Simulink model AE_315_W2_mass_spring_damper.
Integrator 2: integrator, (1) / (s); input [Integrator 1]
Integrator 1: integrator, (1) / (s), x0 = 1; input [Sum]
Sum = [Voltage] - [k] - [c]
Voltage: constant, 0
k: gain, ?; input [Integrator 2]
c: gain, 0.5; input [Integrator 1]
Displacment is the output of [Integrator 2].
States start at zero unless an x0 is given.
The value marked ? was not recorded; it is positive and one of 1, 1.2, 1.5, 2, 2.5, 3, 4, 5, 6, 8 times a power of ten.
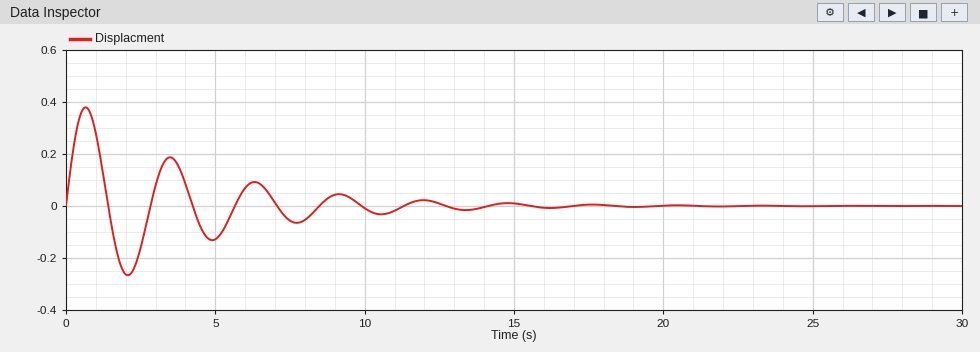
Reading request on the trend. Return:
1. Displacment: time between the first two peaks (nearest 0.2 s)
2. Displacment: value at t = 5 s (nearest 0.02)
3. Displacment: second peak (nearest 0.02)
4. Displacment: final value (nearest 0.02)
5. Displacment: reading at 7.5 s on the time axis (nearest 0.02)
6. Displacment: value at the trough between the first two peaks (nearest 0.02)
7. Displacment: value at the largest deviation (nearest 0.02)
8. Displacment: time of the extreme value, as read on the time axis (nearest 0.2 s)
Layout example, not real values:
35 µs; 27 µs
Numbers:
2.8 s; -0.12; 0.18; 0.00; -0.06; -0.26; 0.38; 0.6 s
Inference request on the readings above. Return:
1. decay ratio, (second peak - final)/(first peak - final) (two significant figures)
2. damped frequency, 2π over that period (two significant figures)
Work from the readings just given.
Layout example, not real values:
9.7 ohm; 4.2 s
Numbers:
0.47; 2.2 rad/s
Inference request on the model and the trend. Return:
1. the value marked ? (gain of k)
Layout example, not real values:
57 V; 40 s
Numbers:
5
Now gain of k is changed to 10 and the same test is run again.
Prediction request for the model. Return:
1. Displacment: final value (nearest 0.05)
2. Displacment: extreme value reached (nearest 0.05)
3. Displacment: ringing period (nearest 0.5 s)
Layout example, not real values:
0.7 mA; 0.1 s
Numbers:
0.00; 0.30; 2.0 s
